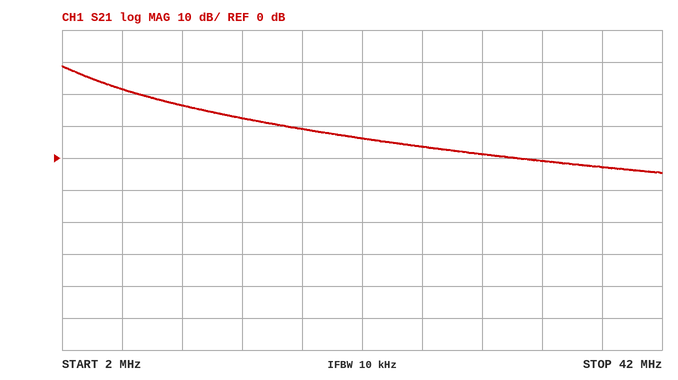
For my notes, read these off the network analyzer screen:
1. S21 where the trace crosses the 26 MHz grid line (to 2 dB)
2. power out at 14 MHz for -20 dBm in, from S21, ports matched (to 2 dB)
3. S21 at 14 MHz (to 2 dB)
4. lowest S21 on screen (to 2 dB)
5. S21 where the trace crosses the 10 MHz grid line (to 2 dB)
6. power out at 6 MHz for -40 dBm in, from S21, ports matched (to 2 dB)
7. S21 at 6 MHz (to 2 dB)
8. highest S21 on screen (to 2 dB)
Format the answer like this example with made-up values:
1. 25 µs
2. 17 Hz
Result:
1. 4 dB
2. -8 dBm
3. 12 dB
4. -4 dB
5. 16 dB
6. -18 dBm
7. 22 dB
8. 28 dB
